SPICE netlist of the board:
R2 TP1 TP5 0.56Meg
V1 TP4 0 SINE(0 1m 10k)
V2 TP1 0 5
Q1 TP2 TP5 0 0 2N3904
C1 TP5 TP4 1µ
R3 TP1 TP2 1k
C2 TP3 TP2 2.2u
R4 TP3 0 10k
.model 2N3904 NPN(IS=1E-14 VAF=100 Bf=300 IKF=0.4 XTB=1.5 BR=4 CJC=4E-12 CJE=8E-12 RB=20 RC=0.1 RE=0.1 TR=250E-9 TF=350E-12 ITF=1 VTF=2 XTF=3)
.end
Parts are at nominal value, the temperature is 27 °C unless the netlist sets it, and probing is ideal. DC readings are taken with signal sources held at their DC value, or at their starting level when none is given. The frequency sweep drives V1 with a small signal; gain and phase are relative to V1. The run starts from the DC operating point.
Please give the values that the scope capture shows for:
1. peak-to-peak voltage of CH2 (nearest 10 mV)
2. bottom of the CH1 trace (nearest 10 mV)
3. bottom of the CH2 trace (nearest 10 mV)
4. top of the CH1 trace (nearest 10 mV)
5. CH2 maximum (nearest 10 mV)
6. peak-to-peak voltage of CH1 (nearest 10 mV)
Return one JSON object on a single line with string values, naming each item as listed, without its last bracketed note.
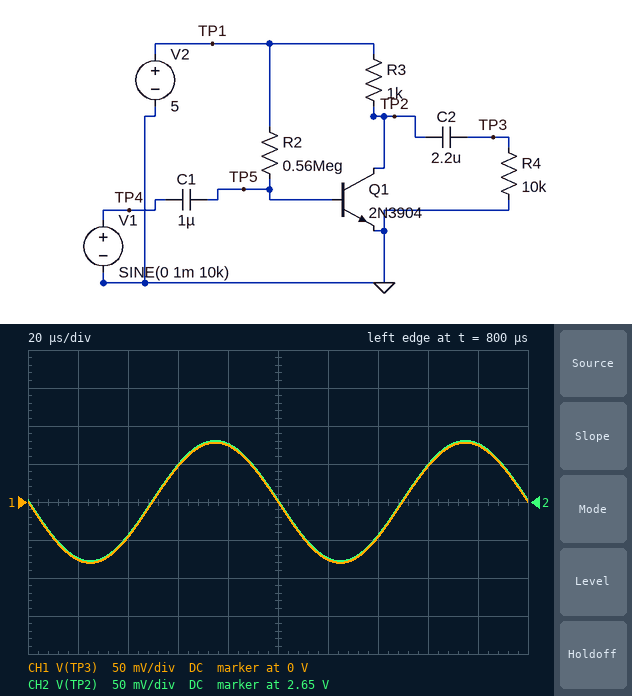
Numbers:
{"peak-to-peak voltage of CH2": "160 mV", "bottom of the CH1 trace": "-80 mV", "bottom of the CH2 trace": "2.57 V", "top of the CH1 trace": "80 mV", "CH2 maximum": "2.73 V", "peak-to-peak voltage of CH1": "160 mV"}
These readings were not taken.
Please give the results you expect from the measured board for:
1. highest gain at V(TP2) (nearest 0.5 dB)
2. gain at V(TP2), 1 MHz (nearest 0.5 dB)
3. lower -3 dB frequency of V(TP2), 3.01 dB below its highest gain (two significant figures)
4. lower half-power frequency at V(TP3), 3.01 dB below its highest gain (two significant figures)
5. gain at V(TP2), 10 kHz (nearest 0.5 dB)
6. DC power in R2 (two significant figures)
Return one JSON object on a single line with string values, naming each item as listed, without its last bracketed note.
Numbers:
{"highest gain at V(TP2)": "38.0 dB", "gain at V(TP2), 1 MHz": "38.0 dB", "lower -3 dB frequency of V(TP2), 3.01 dB below its highest gain": "47 Hz", "lower half-power frequency at V(TP3), 3.01 dB below its highest gain": "48 Hz", "gain at V(TP2), 10 kHz": "38.0 dB", "DC power in R2": "33 µW"}
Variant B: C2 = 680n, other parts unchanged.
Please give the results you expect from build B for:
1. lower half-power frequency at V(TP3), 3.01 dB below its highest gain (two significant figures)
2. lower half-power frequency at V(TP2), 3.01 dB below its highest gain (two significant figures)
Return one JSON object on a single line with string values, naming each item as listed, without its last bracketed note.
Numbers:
{"lower half-power frequency at V(TP3), 3.01 dB below its highest gain": "55 Hz", "lower half-power frequency at V(TP2), 3.01 dB below its highest gain": "45 Hz"}
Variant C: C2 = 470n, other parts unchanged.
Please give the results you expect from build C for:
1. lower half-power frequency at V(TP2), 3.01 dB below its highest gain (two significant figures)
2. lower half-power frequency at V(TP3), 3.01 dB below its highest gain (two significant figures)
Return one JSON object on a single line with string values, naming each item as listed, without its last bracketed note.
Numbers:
{"lower half-power frequency at V(TP2), 3.01 dB below its highest gain": "44 Hz", "lower half-power frequency at V(TP3), 3.01 dB below its highest gain": "61 Hz"}
